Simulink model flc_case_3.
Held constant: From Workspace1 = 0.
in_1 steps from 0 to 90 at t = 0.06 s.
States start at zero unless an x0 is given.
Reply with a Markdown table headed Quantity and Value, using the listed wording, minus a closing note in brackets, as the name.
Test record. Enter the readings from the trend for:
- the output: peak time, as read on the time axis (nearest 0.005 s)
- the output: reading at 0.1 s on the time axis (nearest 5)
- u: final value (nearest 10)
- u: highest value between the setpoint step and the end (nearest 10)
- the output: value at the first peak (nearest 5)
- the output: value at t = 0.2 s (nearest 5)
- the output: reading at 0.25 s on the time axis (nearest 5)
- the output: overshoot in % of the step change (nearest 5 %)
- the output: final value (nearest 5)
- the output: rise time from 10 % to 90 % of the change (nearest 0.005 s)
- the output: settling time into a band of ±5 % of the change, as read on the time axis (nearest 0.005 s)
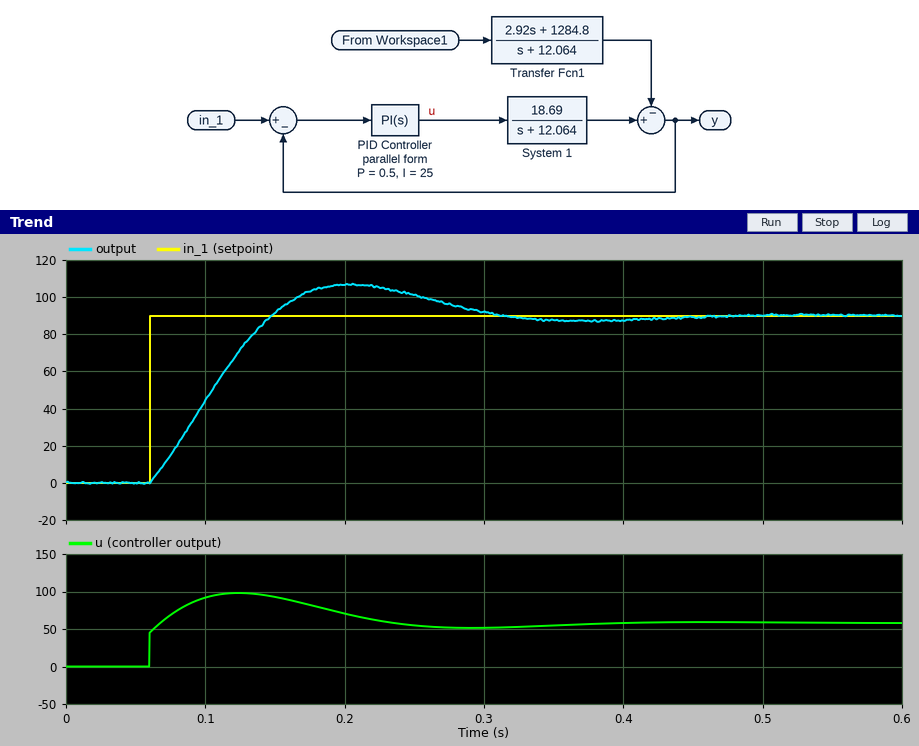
| Quantity | Value |
|---|---|
| the output: peak time, as read on the time axis | 0.205 s |
| the output: reading at 0.1 s on the time axis | 45 |
| u: final value | 60 |
| u: highest value between the setpoint step and the end | 100 |
| the output: value at the first peak | 105 |
| the output: value at t = 0.2 s | 105 |
| the output: reading at 0.25 s on the time axis | 100 |
| the output: overshoot in % of the step change | 20 % |
| the output: final value | 90 |
| the output: rise time from 10 % to 90 % of the change | 0.065 s |
| the output: settling time into a band of ±5 % of the change, as read on the time axis | 0.285 s |
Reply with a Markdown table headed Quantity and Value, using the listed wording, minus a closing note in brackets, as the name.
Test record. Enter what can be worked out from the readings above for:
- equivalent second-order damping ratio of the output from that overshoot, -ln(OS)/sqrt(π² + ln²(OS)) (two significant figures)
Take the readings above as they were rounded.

| Quantity | Value |
|---|---|
| equivalent second-order damping ratio of the output from that overshoot, -ln(OS)/sqrt(π² + ln²(OS)) | 0.46 |
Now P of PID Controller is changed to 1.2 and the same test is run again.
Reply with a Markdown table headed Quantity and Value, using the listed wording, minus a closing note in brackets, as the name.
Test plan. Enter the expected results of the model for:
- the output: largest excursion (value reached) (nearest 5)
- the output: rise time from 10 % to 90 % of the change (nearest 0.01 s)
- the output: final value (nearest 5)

| Quantity | Value |
|---|---|
| the output: largest excursion (value reached) | 95 |
| the output: rise time from 10 % to 90 % of the change | 0.06 s |
| the output: final value | 90 |
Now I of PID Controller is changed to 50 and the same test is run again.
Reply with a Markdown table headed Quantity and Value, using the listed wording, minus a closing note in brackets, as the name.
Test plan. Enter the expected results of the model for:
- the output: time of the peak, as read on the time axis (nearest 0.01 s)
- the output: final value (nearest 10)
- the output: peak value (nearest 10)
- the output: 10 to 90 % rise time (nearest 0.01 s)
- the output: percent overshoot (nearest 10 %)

| Quantity | Value |
|---|---|
| the output: time of the peak, as read on the time axis | 0.16 s |
| the output: final value | 90 |
| the output: peak value | 120 |
| the output: 10 to 90 % rise time | 0.04 s |
| the output: percent overshoot | 30 % |
